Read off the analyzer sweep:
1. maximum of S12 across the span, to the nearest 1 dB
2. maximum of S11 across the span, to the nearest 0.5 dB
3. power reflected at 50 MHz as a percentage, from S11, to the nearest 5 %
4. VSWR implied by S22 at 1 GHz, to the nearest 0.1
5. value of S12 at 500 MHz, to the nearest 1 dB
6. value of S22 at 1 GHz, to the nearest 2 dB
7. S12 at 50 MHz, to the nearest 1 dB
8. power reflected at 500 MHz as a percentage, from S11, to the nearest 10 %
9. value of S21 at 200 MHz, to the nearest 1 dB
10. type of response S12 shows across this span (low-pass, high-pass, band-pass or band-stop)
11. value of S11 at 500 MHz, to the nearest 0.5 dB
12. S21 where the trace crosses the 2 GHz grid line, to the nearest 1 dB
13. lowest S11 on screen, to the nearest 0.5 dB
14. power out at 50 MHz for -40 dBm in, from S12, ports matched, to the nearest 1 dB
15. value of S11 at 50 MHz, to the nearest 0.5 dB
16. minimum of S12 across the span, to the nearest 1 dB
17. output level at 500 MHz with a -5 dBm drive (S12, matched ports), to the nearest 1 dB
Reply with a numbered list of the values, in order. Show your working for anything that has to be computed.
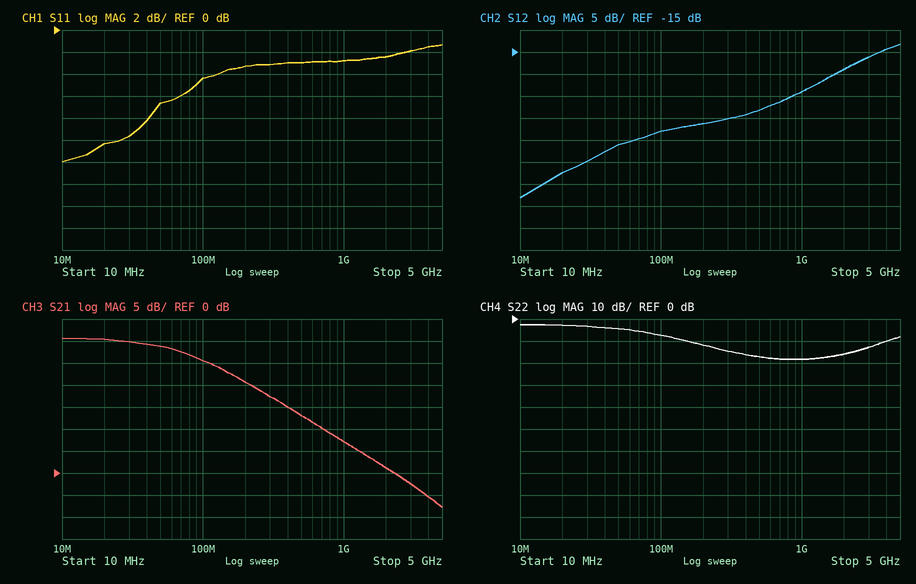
1. -13 dB
2. -1.5 dB
3. 10^(-6.5/10) ≈ 22.4 %, so 20 % to the nearest 5 %
4. |Γ| = 10^(-18/20) = 0.1259; VSWR = (1 + 0.1259)/(1 − 0.1259) ≈ 1.3
5. -28 dB
6. -18 dB
7. -36 dB
8. 10^(-3/10) ≈ 50 %
9. 21 dB
10. high-pass
11. -3.0 dB
12. 1 dB
13. -12.0 dB
14. -40 dBm + (-36 dB) = -76 dBm
15. -6.5 dB
16. -48 dB
17. -5 dBm + (-28 dB) = -33 dBm
